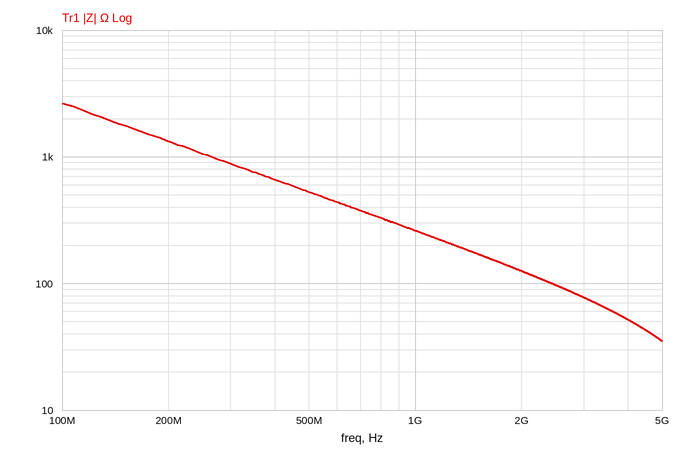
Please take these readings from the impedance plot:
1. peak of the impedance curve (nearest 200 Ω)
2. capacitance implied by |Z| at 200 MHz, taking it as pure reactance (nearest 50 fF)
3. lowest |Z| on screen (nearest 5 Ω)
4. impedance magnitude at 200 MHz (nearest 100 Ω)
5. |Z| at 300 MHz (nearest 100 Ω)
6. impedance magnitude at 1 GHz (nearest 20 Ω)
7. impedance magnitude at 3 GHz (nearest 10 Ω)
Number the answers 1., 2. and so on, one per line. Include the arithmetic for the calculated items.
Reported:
1. 2.6 kΩ
2. C = 1/(2π × 200 MHz × 1.3 kΩ) ≈ 612 fF, so 600 fF to the nearest 50 fF
3. 35 Ω
4. 1.3 kΩ
5. 900 Ω
6. 260 Ω
7. 80 Ω
